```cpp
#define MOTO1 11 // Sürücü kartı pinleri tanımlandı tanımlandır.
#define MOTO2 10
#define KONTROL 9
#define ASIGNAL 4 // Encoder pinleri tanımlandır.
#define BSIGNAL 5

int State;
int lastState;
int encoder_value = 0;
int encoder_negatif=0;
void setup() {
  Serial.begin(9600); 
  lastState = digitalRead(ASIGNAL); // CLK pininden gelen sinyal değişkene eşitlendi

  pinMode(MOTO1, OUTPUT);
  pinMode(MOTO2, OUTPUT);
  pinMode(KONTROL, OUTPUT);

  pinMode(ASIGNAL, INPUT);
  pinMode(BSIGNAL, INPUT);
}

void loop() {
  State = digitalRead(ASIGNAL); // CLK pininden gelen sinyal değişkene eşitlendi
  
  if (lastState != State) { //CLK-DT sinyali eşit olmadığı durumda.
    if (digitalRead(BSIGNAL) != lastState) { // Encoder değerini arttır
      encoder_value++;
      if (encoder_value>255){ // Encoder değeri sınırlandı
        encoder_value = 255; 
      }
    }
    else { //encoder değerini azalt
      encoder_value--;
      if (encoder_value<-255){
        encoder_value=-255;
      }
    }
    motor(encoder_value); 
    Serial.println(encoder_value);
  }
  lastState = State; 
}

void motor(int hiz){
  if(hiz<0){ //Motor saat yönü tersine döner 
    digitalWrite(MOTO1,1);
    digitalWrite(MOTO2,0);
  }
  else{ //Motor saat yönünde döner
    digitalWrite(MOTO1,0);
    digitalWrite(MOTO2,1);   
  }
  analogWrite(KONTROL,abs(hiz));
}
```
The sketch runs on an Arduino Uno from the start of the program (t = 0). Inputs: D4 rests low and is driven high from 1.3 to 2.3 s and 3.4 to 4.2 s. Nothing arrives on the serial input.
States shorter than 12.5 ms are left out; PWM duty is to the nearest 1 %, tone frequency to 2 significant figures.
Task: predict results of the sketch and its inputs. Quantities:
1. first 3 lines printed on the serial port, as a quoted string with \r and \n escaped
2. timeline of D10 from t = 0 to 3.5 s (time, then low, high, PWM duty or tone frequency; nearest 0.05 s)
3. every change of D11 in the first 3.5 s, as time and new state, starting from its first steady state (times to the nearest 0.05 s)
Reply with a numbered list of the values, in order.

1. "-1\r\n0\r\n-1\r\n"
2. 0 s low; 2.3 s high; 3.4 s low
3. 0 s low; 1.3 s high; 2.3 s low; 3.4 s high
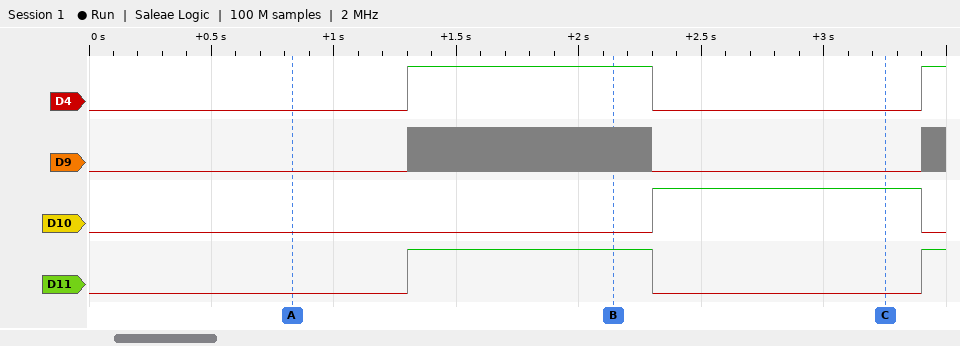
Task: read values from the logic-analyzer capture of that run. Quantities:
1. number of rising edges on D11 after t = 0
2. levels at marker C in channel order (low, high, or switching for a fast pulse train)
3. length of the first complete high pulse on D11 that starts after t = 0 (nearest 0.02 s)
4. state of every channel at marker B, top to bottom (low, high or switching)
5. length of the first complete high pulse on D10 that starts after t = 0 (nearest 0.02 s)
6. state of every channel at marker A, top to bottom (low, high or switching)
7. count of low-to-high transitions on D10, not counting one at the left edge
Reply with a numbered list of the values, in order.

1. 2
2. D4 low, D9 low, D10 high, D11 low
3. 1.00 s
4. D4 high, D9 switching, D10 low, D11 high
5. 1.10 s
6. D4 low, D9 low, D10 low, D11 low
7. 1
